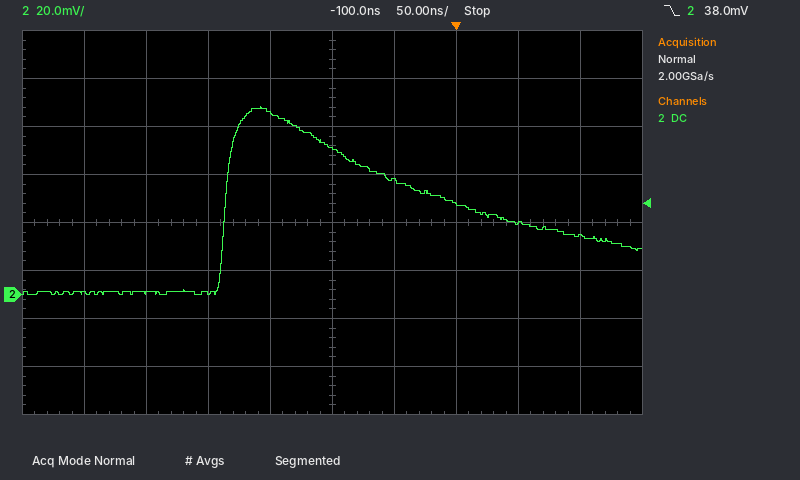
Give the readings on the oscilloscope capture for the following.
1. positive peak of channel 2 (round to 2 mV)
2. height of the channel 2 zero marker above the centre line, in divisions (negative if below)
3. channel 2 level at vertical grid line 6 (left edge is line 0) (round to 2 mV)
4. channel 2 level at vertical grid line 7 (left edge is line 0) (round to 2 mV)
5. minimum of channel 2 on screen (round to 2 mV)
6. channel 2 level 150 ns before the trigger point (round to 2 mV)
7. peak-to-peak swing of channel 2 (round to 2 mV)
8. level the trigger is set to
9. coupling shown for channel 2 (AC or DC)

78 mV
-1.5 div
48 mV
38 mV
0 mV
76 mV
78 mV
38.0 mV
DC
